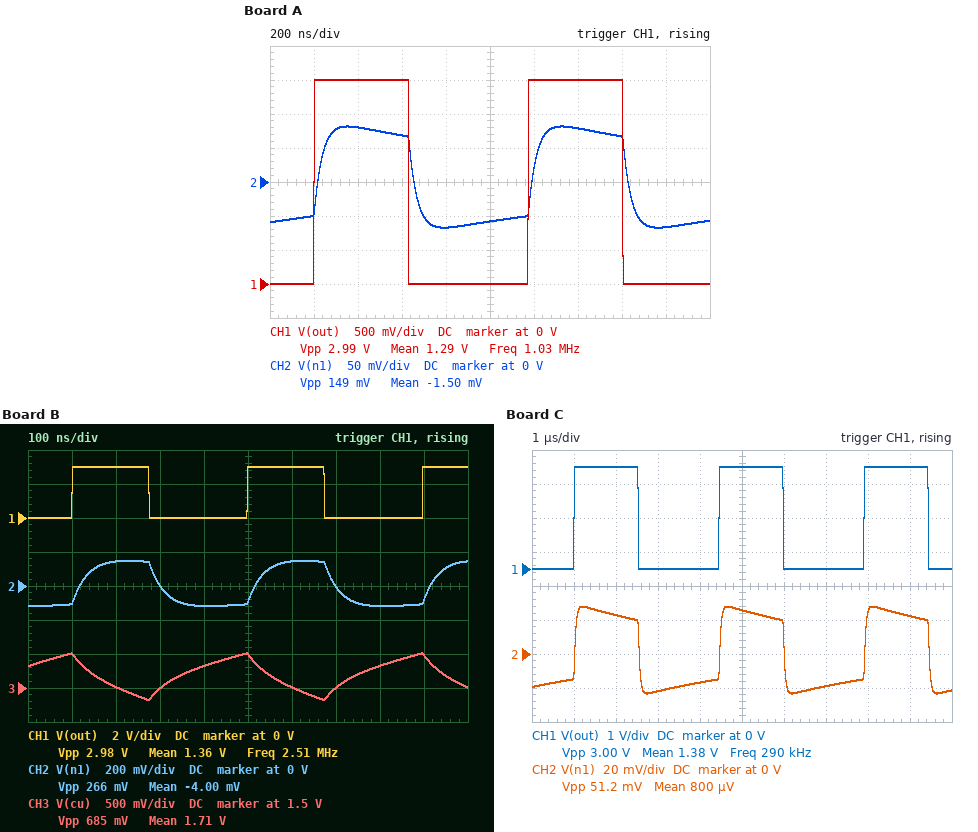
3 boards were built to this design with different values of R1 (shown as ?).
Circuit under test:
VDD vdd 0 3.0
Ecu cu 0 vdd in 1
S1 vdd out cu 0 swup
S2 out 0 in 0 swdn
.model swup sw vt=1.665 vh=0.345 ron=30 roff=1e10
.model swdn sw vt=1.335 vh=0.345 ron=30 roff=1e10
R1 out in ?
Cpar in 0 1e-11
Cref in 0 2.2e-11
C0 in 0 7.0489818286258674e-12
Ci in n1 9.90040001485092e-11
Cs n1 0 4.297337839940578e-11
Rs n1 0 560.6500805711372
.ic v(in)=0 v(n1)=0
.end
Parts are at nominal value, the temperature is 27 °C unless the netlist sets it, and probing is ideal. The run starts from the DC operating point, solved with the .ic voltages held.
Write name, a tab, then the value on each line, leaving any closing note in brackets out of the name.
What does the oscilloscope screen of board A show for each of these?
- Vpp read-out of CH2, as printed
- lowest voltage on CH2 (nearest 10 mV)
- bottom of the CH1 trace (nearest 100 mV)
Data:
Vpp read-out of CH2, as printed	149 mV
lowest voltage on CH2	-70 mV
bottom of the CH1 trace	0 V
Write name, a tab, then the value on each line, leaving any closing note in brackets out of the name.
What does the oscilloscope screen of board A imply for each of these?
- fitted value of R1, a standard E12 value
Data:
fitted value of R1, a standard E12 value	8.2 kΩ
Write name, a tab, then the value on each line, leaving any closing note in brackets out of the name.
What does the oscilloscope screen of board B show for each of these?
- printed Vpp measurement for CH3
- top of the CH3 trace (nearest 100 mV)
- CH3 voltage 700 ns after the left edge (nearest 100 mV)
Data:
printed Vpp measurement for CH3	685 mV
top of the CH3 trace	2.0 V
CH3 voltage 700 ns after the left edge	1.5 V
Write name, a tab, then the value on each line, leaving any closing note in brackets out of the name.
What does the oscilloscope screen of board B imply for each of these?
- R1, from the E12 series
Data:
R1, from the E12 series	3.9 kΩ
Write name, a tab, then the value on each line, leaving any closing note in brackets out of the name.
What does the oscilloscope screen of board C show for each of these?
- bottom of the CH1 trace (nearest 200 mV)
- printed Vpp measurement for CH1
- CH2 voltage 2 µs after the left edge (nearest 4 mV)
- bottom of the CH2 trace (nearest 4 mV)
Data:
bottom of the CH1 trace	0 V
printed Vpp measurement for CH1	3.00 V
CH2 voltage 2 µs after the left edge	24 mV
bottom of the CH2 trace	-24 mV
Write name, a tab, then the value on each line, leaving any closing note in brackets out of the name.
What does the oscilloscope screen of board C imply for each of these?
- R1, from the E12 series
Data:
R1, from the E12 series	27 kΩ
